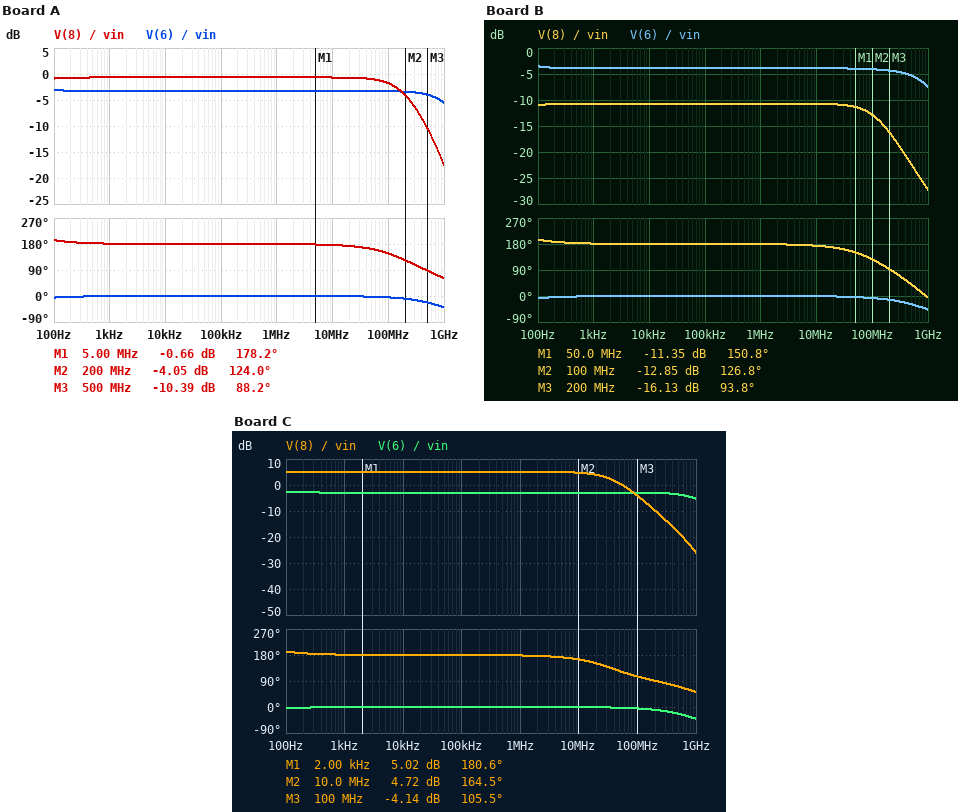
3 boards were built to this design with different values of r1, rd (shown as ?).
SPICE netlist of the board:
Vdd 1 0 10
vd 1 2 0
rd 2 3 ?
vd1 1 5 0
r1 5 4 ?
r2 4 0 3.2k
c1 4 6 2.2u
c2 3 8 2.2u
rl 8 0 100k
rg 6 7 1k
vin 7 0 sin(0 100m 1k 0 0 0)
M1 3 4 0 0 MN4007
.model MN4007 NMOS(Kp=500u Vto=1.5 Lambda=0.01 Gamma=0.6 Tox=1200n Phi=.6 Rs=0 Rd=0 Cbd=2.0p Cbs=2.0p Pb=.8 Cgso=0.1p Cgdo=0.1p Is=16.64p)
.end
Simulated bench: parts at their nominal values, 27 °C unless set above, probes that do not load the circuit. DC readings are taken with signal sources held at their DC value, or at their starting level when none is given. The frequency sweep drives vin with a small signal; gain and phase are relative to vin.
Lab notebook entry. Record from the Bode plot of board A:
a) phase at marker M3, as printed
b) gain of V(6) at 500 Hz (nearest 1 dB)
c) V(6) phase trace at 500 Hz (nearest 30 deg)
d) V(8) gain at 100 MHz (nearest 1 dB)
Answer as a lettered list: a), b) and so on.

a) 88.2 deg
b) -3 dB
c) 0 deg
d) -2 dB
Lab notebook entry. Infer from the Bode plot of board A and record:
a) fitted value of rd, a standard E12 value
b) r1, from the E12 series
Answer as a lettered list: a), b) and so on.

a) 1.5 kΩ
b) 6.8 kΩ
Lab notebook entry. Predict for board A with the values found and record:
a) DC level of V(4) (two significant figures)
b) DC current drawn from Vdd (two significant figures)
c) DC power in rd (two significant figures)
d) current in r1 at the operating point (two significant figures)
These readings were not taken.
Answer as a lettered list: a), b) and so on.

a) 3.2 V
b) 1.8 mA
c) 930 µW
d) 1.0 mA
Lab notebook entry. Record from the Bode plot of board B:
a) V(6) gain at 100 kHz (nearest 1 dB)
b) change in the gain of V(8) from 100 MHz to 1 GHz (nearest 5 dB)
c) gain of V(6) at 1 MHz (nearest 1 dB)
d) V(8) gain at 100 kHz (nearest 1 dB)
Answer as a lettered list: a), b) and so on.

a) -4 dB
b) -15 dB
c) -4 dB
d) -11 dB
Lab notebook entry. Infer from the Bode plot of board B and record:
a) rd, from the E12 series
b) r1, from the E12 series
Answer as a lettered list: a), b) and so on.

a) 6.8 kΩ
b) 3.9 kΩ
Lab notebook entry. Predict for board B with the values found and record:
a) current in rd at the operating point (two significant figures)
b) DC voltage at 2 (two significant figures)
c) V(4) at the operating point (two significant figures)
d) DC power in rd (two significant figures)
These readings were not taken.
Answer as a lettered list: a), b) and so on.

a) 1.3 mA
b) 10 V
c) 4.5 V
d) 12 mW
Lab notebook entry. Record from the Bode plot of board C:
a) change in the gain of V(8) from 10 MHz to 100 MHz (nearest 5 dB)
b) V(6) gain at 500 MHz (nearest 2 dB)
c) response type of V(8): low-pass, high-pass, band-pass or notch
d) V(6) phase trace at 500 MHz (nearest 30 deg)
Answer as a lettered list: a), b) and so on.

a) -10 dB
b) -4 dB
c) low-pass
d) -30 deg
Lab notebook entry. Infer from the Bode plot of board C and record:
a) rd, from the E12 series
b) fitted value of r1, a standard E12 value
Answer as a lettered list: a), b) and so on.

a) 8.2 kΩ
b) 12 kΩ
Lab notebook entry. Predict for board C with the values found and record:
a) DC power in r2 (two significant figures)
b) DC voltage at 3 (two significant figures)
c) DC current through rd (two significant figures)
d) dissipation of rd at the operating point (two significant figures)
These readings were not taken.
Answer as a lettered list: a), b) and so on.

a) 1.4 mW
b) 9.2 V
c) 100 µA
d) 82 µW
